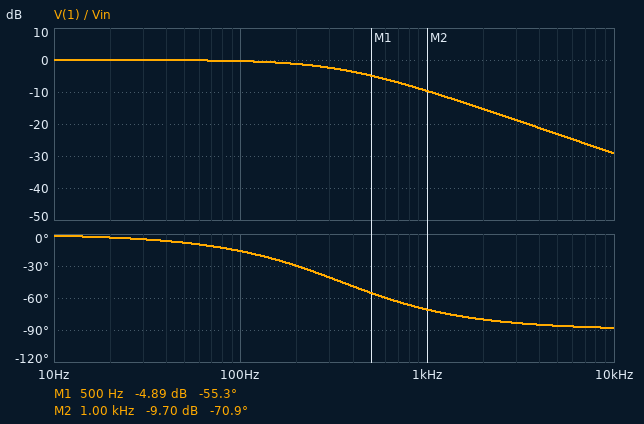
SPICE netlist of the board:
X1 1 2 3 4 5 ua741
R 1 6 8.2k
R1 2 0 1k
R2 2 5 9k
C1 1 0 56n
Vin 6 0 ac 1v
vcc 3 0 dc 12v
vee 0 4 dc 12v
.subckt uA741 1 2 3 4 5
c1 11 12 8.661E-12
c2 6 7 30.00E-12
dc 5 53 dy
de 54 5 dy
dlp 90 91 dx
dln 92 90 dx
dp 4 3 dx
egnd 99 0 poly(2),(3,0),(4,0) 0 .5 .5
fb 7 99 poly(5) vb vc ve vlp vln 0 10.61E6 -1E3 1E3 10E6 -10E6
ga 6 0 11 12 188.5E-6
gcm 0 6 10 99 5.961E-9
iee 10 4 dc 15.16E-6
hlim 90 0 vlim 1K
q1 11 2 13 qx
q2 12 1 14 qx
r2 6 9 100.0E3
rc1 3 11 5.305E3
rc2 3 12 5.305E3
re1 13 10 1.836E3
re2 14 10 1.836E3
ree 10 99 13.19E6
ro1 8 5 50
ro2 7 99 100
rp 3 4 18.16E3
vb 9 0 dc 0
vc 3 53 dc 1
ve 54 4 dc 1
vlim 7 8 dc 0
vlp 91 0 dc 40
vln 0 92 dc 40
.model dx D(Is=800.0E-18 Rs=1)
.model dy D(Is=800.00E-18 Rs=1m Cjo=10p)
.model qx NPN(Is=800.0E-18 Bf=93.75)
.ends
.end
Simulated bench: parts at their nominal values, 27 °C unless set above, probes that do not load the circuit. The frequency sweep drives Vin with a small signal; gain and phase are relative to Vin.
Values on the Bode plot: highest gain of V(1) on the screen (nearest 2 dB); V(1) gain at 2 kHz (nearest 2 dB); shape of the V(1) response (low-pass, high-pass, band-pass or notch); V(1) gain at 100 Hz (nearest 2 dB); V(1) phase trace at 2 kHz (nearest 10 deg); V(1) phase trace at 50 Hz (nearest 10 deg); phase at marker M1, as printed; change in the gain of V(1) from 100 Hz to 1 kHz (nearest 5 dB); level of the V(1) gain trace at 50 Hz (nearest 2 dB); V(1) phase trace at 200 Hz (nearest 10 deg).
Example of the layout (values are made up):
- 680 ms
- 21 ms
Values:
- 0 dB
- -16 dB
- low-pass
- 0 dB
- -80 deg
- -10 deg
- -55.3 deg
- -10 dB
- 0 dB
- -30 deg
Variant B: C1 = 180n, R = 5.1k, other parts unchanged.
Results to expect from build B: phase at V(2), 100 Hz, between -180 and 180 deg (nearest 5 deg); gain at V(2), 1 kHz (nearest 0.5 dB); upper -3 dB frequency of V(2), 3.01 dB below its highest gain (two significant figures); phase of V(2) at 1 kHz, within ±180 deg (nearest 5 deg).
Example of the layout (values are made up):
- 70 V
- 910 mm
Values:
- -30 deg
- -15.5 dB
- 170 Hz
- -80 deg
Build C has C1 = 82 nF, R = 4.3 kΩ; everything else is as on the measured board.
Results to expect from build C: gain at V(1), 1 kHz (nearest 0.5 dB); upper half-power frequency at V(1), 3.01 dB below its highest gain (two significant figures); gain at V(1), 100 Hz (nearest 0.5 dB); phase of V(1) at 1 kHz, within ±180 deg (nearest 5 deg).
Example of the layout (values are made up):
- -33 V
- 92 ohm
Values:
- -7.5 dB
- 450 Hz
- 0 dB
- -65 deg
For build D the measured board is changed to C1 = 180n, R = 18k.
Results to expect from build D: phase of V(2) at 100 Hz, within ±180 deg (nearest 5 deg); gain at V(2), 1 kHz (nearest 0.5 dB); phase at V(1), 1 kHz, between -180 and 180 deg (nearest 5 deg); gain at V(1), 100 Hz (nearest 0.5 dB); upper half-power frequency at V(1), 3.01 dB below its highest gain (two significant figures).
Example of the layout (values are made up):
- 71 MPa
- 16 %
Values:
- -65 deg
- -26.0 dB
- -85 deg
- -7.0 dB
- 49 Hz
